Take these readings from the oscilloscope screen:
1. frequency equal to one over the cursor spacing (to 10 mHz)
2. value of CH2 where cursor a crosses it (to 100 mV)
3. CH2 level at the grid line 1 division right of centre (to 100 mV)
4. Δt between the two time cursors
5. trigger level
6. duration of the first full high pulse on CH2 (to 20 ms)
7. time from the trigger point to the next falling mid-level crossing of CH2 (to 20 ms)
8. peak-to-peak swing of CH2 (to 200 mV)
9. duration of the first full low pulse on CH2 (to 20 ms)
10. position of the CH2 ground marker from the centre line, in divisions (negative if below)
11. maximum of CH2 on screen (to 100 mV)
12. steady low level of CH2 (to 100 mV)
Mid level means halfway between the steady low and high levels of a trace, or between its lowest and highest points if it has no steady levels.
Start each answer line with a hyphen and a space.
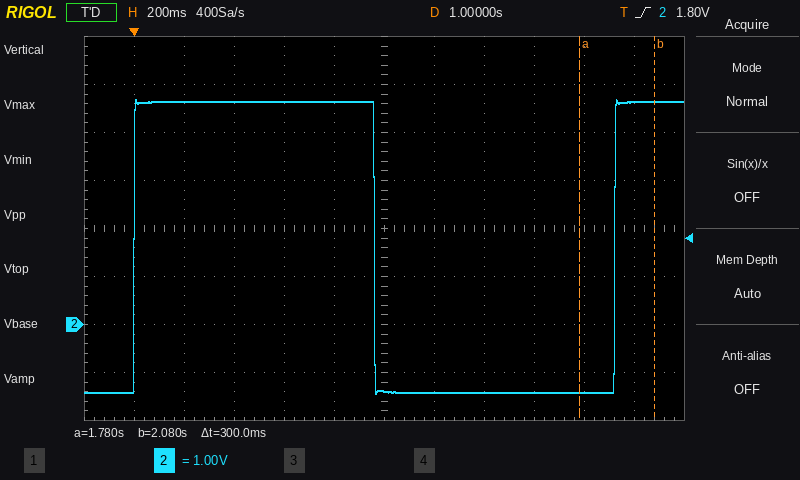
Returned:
- 3.33 Hz
- -1.4 V
- -1.4 V
- 300 ms
- 1.80 V
- 960 ms
- 960 ms
- 6.2 V
- 960 ms
- -2.0 div
- 4.7 V
- -1.4 V
